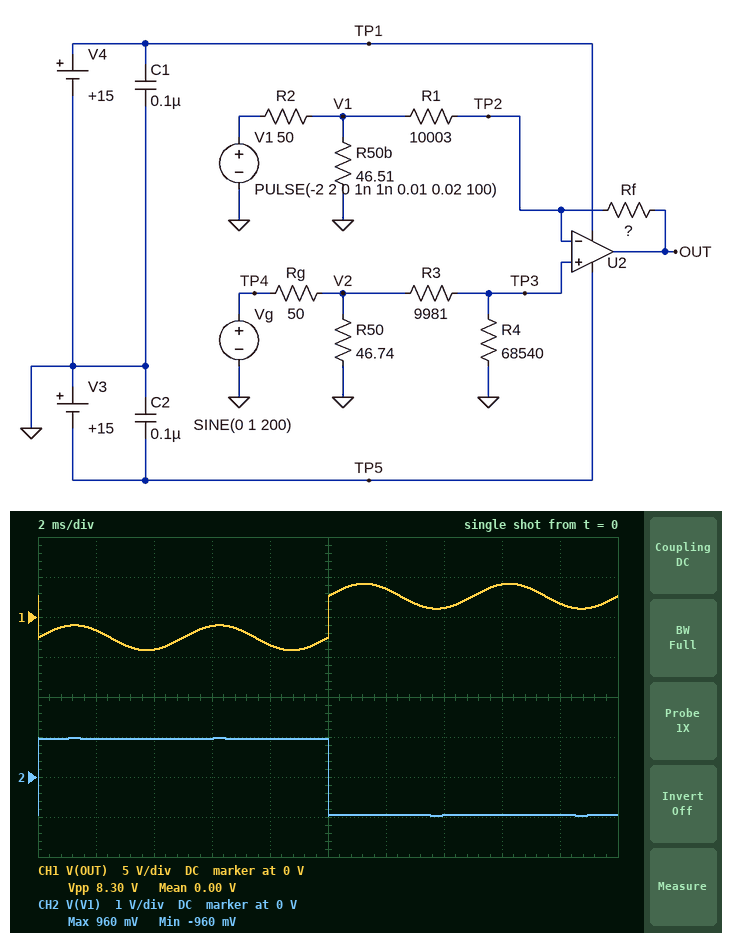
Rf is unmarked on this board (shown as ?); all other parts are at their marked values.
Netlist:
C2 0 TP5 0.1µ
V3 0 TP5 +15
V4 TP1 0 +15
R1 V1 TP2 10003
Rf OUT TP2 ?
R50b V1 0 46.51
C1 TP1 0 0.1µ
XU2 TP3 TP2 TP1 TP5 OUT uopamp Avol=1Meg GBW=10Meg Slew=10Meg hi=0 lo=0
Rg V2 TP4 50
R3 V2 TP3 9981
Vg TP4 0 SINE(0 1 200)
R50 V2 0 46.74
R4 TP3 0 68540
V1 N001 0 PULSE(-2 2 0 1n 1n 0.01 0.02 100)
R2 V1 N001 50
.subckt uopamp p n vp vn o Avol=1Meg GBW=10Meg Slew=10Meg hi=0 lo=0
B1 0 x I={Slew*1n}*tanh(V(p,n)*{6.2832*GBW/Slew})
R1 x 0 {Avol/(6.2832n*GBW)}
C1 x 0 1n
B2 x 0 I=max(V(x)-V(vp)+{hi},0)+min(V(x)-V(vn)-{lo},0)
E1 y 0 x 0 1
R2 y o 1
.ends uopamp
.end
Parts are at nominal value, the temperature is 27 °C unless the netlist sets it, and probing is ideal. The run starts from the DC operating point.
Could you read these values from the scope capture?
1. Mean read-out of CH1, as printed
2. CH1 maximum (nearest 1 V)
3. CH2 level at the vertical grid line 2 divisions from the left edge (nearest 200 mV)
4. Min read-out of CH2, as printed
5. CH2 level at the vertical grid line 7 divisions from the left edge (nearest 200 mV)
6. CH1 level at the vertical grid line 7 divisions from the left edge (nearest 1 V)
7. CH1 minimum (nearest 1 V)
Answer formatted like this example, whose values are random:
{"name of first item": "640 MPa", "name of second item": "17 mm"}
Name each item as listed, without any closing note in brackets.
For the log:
{"Mean read-out of CH1, as printed": "0.00 V", "CH1 maximum": "4 V", "CH2 level at the vertical grid line 2 divisions from the left edge": "1.0 V", "Min read-out of CH2, as printed": "-960 mV", "CH2 level at the vertical grid line 7 divisions from the left edge": "-1.0 V", "CH1 level at the vertical grid line 7 divisions from the left edge": "1 V", "CH1 minimum": "-4 V"}
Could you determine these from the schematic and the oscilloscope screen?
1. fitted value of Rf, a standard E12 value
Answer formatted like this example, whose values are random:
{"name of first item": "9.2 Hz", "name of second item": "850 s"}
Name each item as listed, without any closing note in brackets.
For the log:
{"fitted value of Rf, a standard E12 value": "27 kΩ"}
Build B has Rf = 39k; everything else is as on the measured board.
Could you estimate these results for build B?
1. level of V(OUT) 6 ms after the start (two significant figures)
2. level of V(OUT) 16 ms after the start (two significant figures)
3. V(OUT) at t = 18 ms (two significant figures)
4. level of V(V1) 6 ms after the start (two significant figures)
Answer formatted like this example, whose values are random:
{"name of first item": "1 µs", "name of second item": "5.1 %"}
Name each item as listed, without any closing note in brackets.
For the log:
{"level of V(OUT) 6 ms after the start": "-1.8 V", "level of V(OUT) 16 ms after the start": "5.7 V", "V(OUT) at t = 18 ms": "2.5 V", "level of V(V1) 6 ms after the start": "960 mV"}
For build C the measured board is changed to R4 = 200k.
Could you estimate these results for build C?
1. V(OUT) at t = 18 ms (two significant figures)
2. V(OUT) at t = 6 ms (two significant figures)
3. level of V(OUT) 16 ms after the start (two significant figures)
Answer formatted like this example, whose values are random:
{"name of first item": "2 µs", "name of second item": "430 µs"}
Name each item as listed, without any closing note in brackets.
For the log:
{"V(OUT) at t = 18 ms": "1.6 V", "V(OUT) at t = 6 ms": "-980 mV", "level of V(OUT) 16 ms after the start": "4.2 V"}
